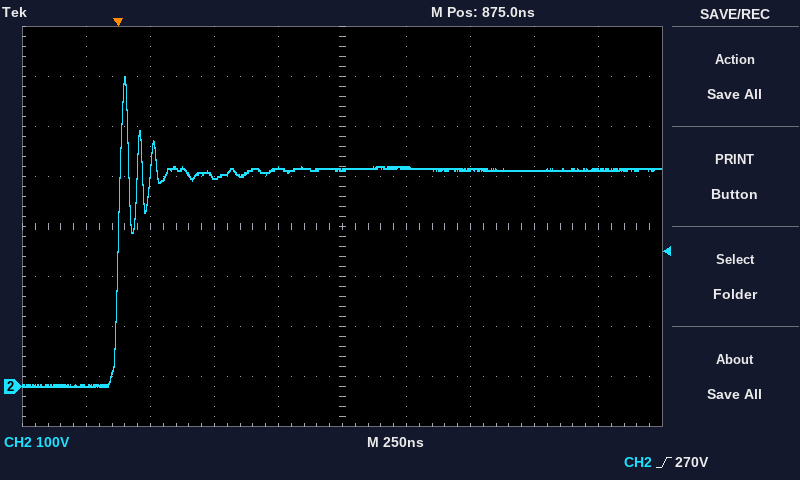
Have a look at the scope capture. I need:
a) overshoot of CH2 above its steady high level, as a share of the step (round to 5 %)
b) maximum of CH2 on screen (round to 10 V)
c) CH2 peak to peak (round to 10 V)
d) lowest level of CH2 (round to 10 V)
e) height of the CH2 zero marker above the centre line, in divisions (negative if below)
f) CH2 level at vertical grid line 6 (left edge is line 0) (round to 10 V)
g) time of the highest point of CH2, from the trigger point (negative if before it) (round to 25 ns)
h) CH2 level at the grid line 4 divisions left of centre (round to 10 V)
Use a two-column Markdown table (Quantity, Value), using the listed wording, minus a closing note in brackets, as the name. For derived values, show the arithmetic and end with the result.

| Quantity | Value |
|---|---|
| overshoot of CH2 above its steady high level, as a share of the step | 45 % |
| maximum of CH2 on screen | 620 V |
| CH2 peak to peak | 620 V − (0 V) = 620 V |
| lowest level of CH2 | 0 V |
| height of the CH2 zero marker above the centre line, in divisions | -3.2 div |
| CH2 level at vertical grid line 6 (left edge is line 0) | 440 V |
| time of the highest point of CH2, from the trigger point (negative if before it) | +25 ns |
| CH2 level at the grid line 4 divisions left of centre | 0 V |
